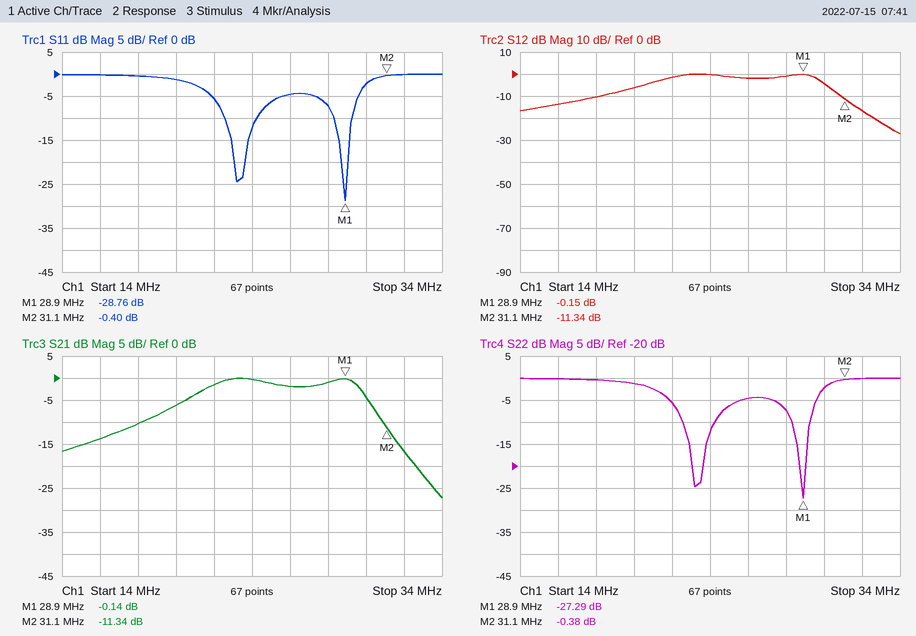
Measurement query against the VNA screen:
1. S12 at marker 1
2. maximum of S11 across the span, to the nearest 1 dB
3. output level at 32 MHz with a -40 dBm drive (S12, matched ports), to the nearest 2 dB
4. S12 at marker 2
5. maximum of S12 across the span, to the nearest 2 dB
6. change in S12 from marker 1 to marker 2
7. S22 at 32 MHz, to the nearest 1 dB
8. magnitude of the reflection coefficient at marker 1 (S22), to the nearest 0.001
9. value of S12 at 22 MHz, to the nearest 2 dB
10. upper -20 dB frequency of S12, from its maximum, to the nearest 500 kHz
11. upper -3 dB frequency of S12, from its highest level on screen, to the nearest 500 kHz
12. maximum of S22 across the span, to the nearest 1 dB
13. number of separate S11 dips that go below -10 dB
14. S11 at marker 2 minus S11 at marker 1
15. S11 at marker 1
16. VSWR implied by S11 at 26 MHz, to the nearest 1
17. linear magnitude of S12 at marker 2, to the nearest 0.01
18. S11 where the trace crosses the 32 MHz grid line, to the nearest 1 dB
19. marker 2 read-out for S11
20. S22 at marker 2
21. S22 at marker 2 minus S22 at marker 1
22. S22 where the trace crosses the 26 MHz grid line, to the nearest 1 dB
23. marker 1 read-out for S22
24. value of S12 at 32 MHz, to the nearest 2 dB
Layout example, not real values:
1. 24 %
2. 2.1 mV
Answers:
1. -0.15 dB
2. 0 dB
3. -56 dBm
4. -11.34 dB
5. 0 dB
6. -11.19 dB
7. 0 dB
8. 0.043
9. -2 dB
10. 32.5 MHz
11. 30.0 MHz
12. 0 dB
13. 2
14. 28.36 dB
15. -28.76 dB
16. 4
17. 0.27
18. 0 dB
19. -0.40 dB
20. -0.38 dB
21. 26.91 dB
22. -5 dB
23. -27.29 dB
24. -16 dB
